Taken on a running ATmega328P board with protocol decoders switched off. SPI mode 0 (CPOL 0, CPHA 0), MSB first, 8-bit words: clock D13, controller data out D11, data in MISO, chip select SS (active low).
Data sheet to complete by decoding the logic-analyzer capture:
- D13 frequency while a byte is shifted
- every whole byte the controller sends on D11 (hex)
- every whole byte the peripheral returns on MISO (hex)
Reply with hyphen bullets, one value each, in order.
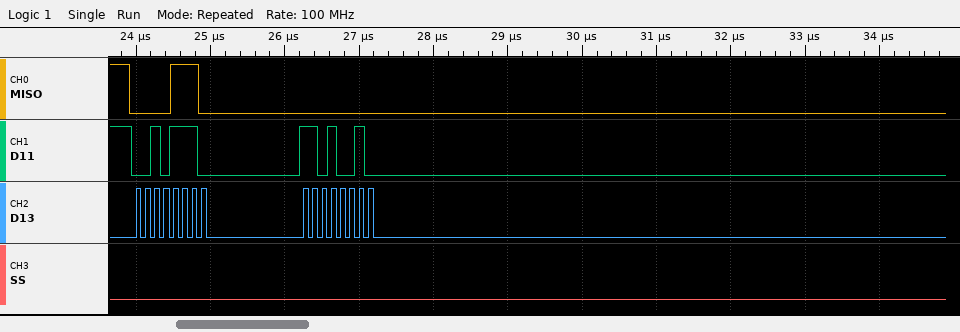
- 8 MHz
- 0x2E 0xD2
- 0x0E 0x00
